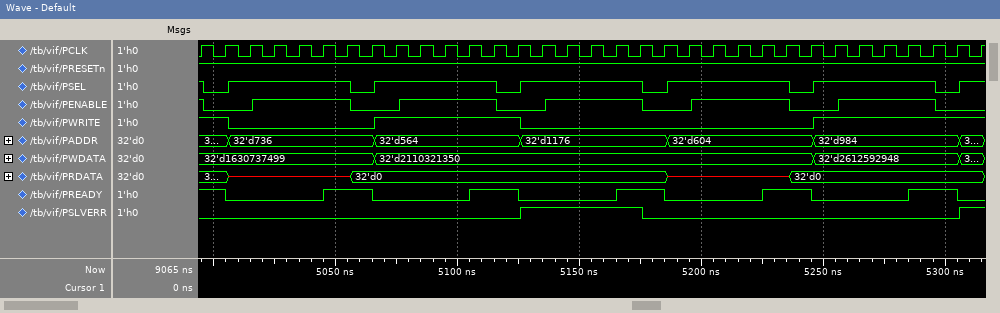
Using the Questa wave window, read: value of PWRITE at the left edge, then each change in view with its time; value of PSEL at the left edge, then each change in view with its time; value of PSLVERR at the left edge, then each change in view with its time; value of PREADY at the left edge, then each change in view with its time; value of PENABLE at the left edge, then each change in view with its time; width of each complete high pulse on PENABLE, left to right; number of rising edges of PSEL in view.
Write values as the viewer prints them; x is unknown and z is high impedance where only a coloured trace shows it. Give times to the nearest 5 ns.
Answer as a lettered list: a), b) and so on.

a) 1, 0 at 5005 ns, 1 at 5065 ns, 0 at 5125 ns, 1 at 5245 ns
b) 1, 0 at 4995 ns, 1 at 5005 ns, 0 at 5055 ns, 1 at 5065 ns, 0 at 5115 ns, 1 at 5125 ns, 0 at 5175 ns, 1 at 5185 ns, 0 at 5235 ns, 1 at 5245 ns, 0 at 5295 ns, 1 at 5305 ns
c) 0, 1 at 5125 ns, 0 at 5175 ns, 1 at 5305 ns
d) 1, 0 at 5005 ns, 1 at 5045 ns, 0 at 5065 ns, 1 at 5105 ns, 0 at 5125 ns, 1 at 5165 ns, 0 at 5185 ns, 1 at 5225 ns, 0 at 5245 ns, 1 at 5285 ns, 0 at 5305 ns
e) 1, 0 at 4995 ns, 1 at 5015 ns, 0 at 5055 ns, 1 at 5075 ns, 0 at 5115 ns, 1 at 5135 ns, 0 at 5175 ns, 1 at 5195 ns, 0 at 5235 ns, 1 at 5255 ns, 0 at 5295 ns
f) 40 ns, 40 ns, 40 ns, 40 ns, 40 ns
g) 6
